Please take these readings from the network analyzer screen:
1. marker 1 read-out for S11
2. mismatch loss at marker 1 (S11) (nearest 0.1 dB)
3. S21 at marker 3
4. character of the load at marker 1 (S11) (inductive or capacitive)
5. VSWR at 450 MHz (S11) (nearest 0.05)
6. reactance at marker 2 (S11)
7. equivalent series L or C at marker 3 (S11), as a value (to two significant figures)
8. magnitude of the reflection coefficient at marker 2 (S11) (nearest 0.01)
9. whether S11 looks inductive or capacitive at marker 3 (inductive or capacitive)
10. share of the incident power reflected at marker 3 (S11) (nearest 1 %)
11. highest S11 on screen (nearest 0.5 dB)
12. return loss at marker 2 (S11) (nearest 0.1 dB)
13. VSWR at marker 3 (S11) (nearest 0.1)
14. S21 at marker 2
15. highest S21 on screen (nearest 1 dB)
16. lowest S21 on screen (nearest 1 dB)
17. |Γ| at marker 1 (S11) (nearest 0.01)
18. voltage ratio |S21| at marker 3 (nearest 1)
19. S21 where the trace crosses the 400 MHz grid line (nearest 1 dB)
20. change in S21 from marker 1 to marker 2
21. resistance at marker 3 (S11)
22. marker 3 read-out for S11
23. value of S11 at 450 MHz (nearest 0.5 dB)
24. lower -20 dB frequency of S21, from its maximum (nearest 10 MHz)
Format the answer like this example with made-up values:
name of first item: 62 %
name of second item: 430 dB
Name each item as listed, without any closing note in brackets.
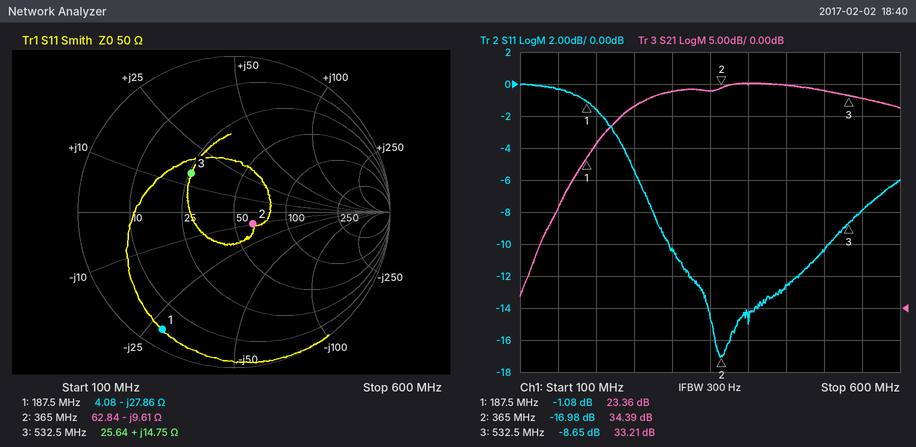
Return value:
marker 1 read-out for S11: -1.08 dB
mismatch loss at marker 1 (S11): 6.6 dB
S21 at marker 3: 33.21 dB
character of the load at marker 1 (S11): capacitive
VSWR at 450 MHz (S11): 1.60
reactance at marker 2: -9.61 Ω
equivalent series L or C at marker 3 (S11), as a value: 4.4 nH
magnitude of the reflection coefficient at marker 2 (S11): 0.14
whether S11 looks inductive or capacitive at marker 3: inductive
share of the incident power reflected at marker 3 (S11): 14 %
highest S11 on screen: 0.0 dB
return loss at marker 2 (S11): 17.0 dB
VSWR at marker 3 (S11): 2.2
S21 at marker 2: 34.39 dB
highest S21 on screen: 35 dB
lowest S21 on screen: 2 dB
|Γ| at marker 1 (S11): 0.88
voltage ratio |S21| at marker 3: 46
S21 where the trace crosses the 400 MHz grid line: 35 dB
change in S21 from marker 1 to marker 2: 11.03 dB
resistance at marker 3: 25.64 Ω
marker 3 read-out for S11: -8.65 dB
value of S11 at 450 MHz: -12.5 dB
lower -20 dB frequency of S21, from its maximum: 150 MHz
